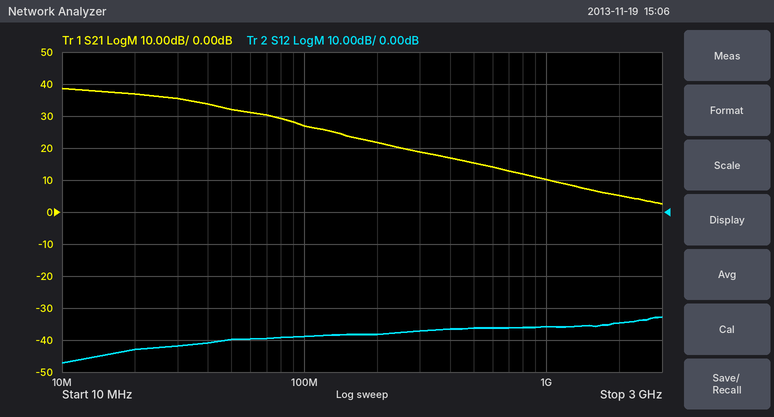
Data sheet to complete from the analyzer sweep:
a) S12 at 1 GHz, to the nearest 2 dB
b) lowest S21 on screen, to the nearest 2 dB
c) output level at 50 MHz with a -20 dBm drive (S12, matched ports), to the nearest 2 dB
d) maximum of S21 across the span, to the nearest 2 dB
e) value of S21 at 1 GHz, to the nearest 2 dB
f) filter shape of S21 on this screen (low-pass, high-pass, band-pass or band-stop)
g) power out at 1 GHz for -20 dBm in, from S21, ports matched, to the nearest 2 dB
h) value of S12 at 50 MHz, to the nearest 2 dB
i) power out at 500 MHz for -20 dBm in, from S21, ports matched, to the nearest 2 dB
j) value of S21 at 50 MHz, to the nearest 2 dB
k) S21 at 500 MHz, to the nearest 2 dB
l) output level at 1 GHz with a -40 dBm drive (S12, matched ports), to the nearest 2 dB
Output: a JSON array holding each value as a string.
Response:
["-36 dB", "2 dB", "-60 dBm", "38 dB", "10 dB", "low-pass", "-10 dBm", "-40 dB", "-4 dBm", "32 dB", "16 dB", "-76 dBm"]
